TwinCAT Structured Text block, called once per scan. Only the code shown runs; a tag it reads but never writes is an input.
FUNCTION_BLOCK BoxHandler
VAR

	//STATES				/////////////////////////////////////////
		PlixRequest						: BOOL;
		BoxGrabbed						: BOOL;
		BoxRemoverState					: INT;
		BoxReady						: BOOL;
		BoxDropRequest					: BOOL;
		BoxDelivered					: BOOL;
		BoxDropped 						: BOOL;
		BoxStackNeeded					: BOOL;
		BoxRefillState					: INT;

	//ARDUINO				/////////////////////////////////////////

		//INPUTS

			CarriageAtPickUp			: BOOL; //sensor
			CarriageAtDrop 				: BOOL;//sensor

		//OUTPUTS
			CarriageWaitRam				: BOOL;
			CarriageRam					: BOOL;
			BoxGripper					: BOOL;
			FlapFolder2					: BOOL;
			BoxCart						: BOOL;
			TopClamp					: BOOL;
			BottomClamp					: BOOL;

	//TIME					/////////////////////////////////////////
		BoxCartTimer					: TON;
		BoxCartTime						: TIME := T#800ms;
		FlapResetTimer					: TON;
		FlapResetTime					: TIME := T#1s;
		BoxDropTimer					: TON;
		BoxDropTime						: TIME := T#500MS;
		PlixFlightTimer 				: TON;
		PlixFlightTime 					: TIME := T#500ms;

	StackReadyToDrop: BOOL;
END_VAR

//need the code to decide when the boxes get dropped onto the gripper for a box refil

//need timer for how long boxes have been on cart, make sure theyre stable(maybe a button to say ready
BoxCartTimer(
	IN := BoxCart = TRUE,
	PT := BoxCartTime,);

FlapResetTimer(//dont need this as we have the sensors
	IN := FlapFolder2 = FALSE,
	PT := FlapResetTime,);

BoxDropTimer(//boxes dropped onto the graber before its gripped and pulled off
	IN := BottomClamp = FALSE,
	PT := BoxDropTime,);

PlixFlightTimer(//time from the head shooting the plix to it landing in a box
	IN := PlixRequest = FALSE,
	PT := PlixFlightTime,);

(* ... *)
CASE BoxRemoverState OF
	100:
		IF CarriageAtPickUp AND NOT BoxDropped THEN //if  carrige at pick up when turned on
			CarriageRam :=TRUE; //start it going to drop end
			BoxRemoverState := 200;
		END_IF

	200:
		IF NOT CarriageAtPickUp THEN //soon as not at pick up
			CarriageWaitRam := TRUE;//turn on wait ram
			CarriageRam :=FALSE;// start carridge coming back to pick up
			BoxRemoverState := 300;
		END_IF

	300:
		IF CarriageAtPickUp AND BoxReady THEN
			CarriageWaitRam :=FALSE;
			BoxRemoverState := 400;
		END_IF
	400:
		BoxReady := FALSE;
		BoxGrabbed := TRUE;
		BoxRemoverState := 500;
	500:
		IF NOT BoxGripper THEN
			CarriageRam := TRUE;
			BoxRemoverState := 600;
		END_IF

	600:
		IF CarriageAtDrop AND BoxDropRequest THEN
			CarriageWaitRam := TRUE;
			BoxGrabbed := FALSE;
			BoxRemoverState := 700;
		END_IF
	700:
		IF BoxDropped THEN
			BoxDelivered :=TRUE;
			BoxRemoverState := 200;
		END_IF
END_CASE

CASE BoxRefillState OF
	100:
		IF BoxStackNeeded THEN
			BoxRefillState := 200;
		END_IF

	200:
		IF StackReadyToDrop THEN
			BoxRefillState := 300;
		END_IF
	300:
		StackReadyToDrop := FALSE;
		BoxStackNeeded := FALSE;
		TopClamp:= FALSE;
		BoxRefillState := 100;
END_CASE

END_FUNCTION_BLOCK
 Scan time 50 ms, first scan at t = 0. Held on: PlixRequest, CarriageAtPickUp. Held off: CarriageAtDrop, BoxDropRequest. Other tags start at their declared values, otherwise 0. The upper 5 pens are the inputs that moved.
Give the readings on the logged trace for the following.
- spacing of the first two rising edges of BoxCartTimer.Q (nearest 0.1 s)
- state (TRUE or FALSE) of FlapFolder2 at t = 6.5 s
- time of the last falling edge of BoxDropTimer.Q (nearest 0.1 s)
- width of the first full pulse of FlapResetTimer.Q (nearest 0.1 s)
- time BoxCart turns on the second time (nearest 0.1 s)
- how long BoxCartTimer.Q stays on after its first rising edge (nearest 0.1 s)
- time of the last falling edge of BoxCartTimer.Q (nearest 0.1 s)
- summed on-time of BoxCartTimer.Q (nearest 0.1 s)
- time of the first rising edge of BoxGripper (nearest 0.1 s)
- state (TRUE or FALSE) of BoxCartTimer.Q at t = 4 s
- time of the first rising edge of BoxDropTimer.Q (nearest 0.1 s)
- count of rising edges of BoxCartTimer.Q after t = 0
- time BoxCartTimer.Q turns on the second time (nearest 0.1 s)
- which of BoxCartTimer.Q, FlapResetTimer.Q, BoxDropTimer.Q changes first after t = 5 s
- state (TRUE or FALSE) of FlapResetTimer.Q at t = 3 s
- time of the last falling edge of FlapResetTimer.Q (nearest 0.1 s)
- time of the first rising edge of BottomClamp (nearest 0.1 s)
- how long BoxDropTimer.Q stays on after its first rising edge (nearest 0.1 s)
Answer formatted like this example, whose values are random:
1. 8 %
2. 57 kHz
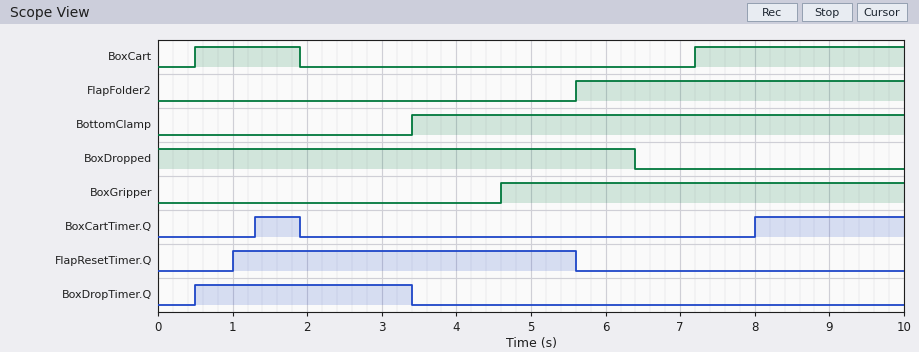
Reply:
1. 6.7 s
2. TRUE
3. 3.4 s
4. 4.6 s
5. 7.2 s
6. 0.6 s
7. 1.9 s
8. 2.6 s
9. 4.6 s
10. FALSE
11. 0.5 s
12. 2
13. 8.0 s
14. FlapResetTimer.Q
15. TRUE
16. 5.6 s
17. 3.4 s
18. 2.9 s
